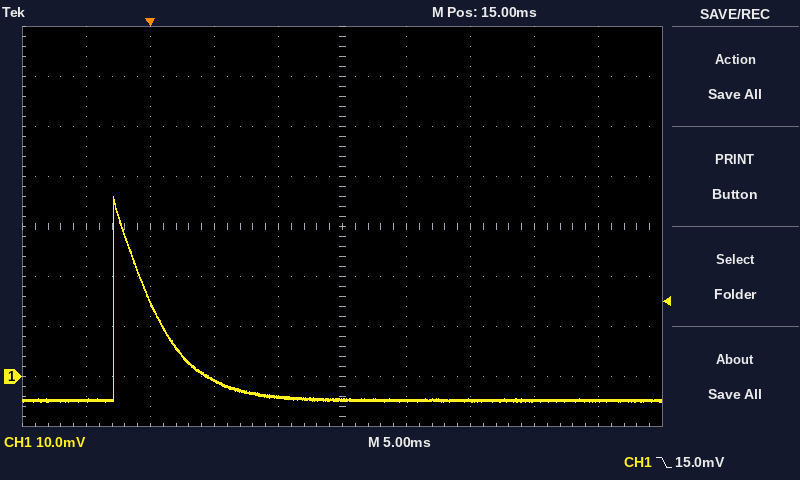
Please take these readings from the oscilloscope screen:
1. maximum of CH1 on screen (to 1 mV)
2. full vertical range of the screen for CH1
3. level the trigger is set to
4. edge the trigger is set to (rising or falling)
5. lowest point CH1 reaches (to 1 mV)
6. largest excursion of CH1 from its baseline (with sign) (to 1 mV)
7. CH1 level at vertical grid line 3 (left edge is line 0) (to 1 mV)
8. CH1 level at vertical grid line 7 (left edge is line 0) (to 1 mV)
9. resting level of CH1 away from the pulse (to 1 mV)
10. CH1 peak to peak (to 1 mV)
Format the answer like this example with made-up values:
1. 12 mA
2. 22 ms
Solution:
1. 36 mV
2. 80 mV
3. 15.0 mV
4. falling
5. -5 mV
6. +41 mV
7. -1 mV
8. -5 mV
9. -5 mV
10. 41 mV
